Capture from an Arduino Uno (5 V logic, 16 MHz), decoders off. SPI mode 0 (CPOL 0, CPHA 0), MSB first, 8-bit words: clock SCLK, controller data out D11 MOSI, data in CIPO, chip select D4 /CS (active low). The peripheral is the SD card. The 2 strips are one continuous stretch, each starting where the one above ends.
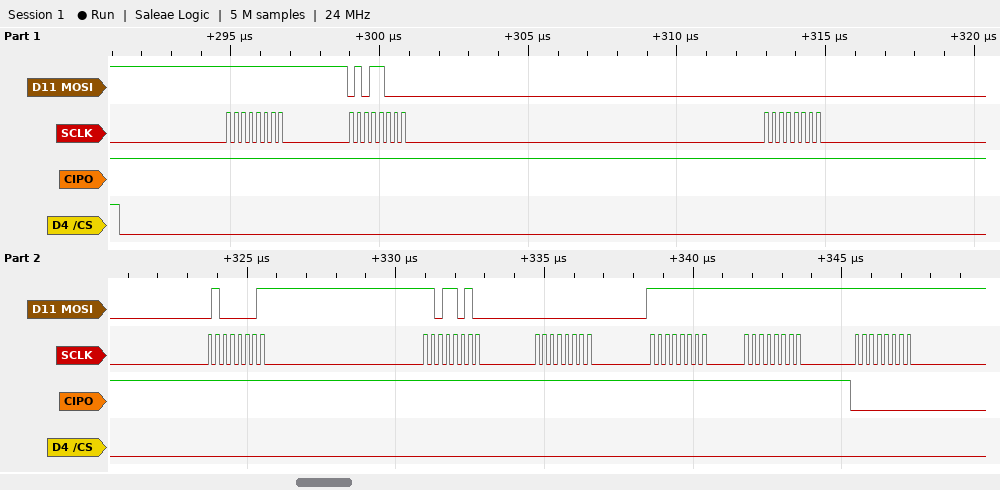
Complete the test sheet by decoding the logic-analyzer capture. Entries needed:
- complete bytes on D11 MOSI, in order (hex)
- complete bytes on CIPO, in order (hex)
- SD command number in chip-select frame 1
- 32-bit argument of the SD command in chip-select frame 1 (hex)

0xFF 0x58 0x00 0x41 0xDA 0x00 0xFF 0xFF 0xFF
0xFF 0xFF 0xFF 0xFF 0xFF 0xFF 0xFF 0xFF 0x00
CMD24
0x0041DA00
